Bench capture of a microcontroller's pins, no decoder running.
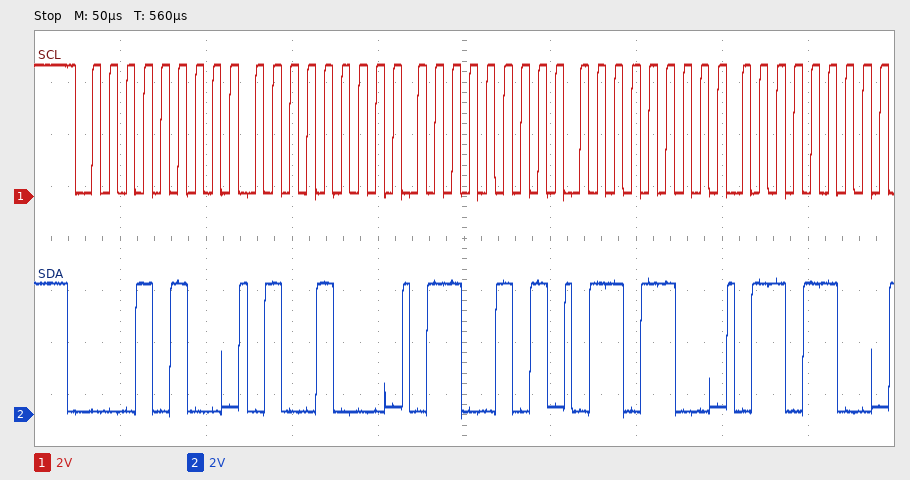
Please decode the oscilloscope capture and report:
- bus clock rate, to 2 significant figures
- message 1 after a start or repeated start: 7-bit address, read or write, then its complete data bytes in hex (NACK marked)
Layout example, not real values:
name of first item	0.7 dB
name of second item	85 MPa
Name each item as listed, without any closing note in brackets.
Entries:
bus clock rate, to 2 significant figures	100 kHz
message 1 after a start or repeated start: 7-bit address, read or write, then its complete data bytes in hex	0x0A write: 48 65 6C 6C
